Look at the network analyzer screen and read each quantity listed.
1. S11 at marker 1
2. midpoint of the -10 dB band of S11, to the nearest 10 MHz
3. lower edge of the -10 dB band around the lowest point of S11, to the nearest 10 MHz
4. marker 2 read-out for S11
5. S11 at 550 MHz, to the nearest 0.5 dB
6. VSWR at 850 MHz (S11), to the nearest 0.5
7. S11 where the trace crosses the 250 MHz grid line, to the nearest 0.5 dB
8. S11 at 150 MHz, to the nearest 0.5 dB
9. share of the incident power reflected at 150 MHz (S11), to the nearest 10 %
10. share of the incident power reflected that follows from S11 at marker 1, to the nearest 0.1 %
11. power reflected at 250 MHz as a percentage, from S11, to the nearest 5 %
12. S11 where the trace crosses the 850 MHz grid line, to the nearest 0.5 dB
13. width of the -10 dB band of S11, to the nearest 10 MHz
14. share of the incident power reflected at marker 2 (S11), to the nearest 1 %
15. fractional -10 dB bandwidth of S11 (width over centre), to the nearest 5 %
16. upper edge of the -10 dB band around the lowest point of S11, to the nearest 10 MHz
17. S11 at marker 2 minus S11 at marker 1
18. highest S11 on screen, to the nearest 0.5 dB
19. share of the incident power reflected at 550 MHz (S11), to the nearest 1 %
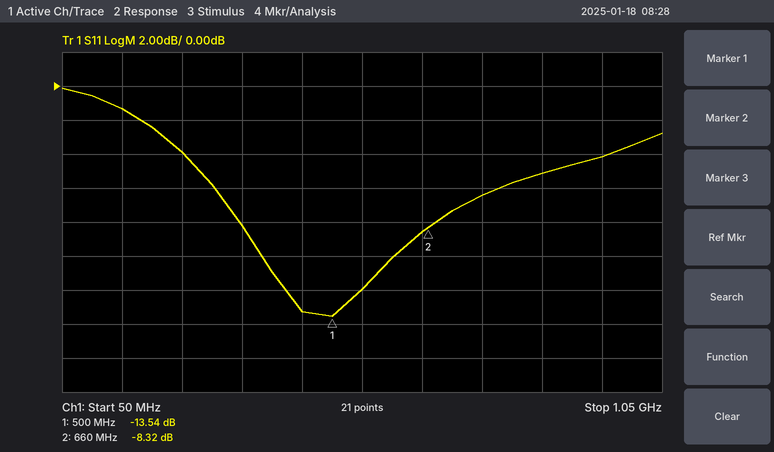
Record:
-13.54 dB
490 MHz
380 MHz
-8.32 dB
-12.0 dB
3.5
-4.0 dB
-1.5 dB
70 %
4.4 %
40 %
-5.0 dB
220 MHz
15 %
45 %
600 MHz
5.22 dB
0.0 dB
6 %
